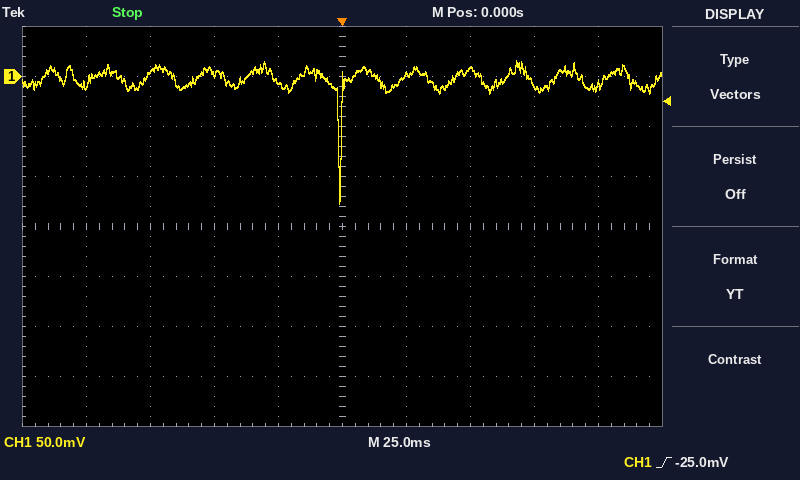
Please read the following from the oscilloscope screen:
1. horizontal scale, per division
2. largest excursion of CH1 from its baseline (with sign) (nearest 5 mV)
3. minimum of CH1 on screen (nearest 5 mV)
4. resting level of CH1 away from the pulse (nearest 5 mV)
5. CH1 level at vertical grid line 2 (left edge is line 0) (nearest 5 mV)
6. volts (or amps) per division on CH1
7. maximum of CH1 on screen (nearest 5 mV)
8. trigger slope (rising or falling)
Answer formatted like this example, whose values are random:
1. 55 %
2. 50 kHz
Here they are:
1. 25 ms
2. -125 mV
3. -125 mV
4. 0 mV
5. 5 mV
6. 50 mV
7. 15 mV
8. rising
